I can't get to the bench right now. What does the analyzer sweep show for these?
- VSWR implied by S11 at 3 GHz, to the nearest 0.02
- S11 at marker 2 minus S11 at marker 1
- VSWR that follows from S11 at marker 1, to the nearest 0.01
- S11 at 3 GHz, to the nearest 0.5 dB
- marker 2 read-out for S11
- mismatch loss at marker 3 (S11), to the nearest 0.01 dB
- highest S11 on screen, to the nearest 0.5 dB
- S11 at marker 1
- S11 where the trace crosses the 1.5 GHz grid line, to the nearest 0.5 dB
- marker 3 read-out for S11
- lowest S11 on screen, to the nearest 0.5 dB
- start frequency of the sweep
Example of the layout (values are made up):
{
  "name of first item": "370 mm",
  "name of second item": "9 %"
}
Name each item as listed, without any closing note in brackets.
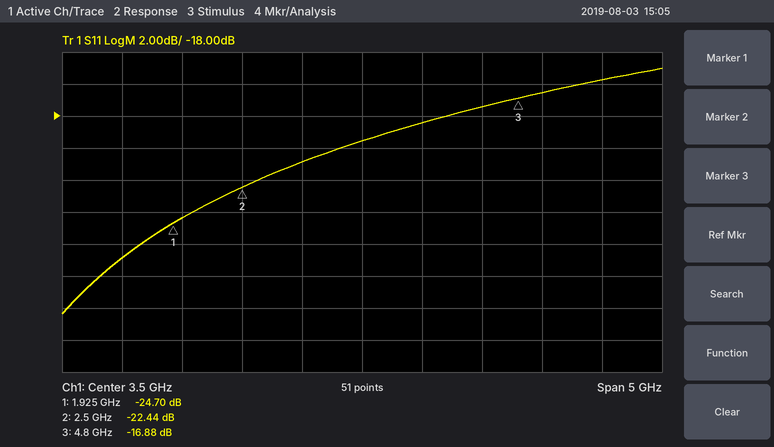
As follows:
{
  "VSWR implied by S11 at 3 GHz, to the nearest 0.02": "1.20",
  "S11 at marker 2 minus S11 at marker 1": "2.26 dB",
  "VSWR that follows from S11 at marker 1, to the nearest 0.01": "1.12",
  "S11 at 3 GHz, to the nearest 0.5 dB": "-21.0 dB",
  "marker 2 read-out for S11": "-22.44 dB",
  "mismatch loss at marker 3 (S11), to the nearest 0.01 dB": "0.09 dB",
  "highest S11 on screen, to the nearest 0.5 dB": "-15.0 dB",
  "S11 at marker 1": "-24.70 dB",
  "S11 where the trace crosses the 1.5 GHz grid line, to the nearest 0.5 dB": "-27.0 dB",
  "marker 3 read-out for S11": "-16.88 dB",
  "lowest S11 on screen, to the nearest 0.5 dB": "-30.5 dB",
  "start frequency of the sweep": "1 GHz"
}
